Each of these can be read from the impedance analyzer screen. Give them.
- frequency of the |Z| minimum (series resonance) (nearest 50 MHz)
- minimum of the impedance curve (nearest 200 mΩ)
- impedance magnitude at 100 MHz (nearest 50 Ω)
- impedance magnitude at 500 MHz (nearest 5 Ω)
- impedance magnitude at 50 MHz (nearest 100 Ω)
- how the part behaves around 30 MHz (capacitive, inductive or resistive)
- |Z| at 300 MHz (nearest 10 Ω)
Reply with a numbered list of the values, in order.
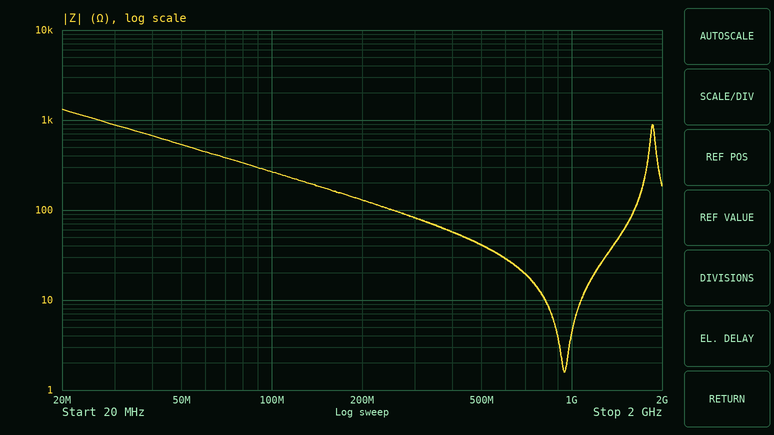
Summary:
1. 950 MHz
2. 1.6 Ω
3. 250 Ω
4. 40 Ω
5. 500 Ω
6. capacitive
7. 80 Ω
